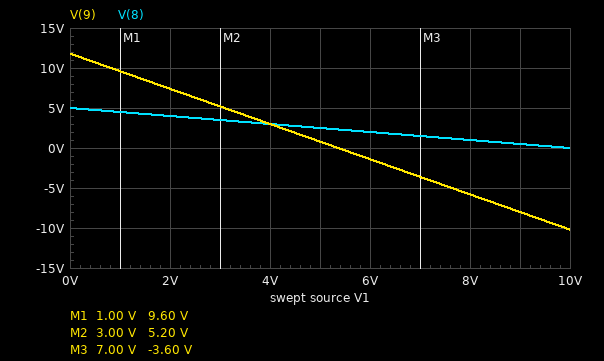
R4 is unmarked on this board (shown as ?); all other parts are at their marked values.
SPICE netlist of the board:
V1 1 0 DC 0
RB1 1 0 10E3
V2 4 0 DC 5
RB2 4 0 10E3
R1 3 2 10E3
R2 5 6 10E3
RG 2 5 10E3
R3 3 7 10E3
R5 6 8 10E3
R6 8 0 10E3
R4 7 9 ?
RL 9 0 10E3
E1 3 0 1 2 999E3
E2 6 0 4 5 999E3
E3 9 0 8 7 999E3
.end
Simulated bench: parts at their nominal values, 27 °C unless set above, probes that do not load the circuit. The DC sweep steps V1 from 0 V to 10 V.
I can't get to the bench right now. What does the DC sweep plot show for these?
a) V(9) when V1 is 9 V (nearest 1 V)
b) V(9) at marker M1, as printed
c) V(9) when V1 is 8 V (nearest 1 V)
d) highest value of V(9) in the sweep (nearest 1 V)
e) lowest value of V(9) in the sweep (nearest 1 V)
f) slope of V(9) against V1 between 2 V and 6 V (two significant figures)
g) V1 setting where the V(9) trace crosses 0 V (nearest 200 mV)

-8 V
9.60 V
-6 V
12 V
-10 V
-2.2 V/V
5.4 V
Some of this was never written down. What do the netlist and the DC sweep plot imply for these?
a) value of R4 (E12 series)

6.8 kΩ
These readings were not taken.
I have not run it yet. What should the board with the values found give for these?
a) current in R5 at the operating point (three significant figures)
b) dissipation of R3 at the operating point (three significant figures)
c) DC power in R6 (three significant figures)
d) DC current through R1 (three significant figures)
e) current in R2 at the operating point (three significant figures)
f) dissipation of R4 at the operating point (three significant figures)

500 µA
10.0 mW
2.50 mW
500 µA
500 µA
6.80 mW
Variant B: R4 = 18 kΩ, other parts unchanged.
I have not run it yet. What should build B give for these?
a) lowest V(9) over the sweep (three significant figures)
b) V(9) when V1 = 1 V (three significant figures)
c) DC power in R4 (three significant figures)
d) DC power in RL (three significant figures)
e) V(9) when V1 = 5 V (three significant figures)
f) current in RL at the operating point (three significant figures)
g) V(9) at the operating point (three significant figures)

-27.0 V
18.0 V
18.0 mW
52.9 mW
-2.00 V
2.30 mA
23.0 V
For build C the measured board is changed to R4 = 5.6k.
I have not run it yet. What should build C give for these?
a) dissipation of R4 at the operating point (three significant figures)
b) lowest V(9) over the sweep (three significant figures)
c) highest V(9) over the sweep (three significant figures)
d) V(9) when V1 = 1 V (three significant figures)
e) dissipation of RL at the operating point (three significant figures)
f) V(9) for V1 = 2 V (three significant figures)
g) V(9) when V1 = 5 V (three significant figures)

5.60 mW
-8.40 V
10.6 V
8.70 V
11.2 mW
6.80 V
1.10 V
